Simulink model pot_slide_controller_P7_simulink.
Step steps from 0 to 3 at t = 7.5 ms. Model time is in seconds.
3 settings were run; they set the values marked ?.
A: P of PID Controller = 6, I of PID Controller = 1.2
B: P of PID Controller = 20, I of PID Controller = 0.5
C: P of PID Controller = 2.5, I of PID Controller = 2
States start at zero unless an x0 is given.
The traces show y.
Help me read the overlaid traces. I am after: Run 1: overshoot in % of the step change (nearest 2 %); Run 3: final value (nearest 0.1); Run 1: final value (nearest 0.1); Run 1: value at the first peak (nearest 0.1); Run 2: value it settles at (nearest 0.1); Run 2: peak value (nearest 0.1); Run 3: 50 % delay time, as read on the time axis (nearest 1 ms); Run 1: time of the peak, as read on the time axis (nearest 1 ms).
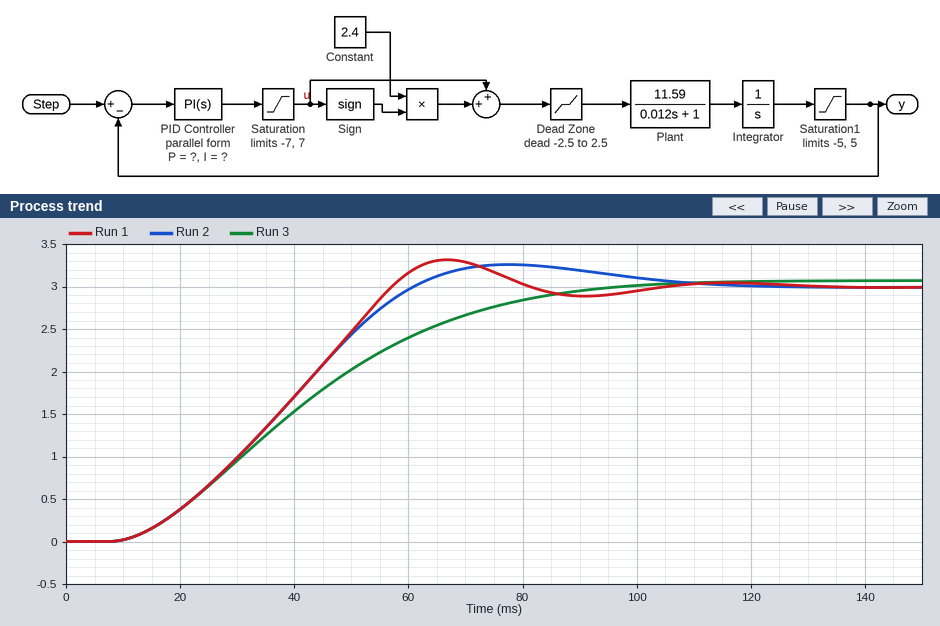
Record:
10 %
3.1
3.0
3.3
3.0
3.3
40 ms
67 ms
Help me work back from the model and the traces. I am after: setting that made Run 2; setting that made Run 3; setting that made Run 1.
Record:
A
C
B
